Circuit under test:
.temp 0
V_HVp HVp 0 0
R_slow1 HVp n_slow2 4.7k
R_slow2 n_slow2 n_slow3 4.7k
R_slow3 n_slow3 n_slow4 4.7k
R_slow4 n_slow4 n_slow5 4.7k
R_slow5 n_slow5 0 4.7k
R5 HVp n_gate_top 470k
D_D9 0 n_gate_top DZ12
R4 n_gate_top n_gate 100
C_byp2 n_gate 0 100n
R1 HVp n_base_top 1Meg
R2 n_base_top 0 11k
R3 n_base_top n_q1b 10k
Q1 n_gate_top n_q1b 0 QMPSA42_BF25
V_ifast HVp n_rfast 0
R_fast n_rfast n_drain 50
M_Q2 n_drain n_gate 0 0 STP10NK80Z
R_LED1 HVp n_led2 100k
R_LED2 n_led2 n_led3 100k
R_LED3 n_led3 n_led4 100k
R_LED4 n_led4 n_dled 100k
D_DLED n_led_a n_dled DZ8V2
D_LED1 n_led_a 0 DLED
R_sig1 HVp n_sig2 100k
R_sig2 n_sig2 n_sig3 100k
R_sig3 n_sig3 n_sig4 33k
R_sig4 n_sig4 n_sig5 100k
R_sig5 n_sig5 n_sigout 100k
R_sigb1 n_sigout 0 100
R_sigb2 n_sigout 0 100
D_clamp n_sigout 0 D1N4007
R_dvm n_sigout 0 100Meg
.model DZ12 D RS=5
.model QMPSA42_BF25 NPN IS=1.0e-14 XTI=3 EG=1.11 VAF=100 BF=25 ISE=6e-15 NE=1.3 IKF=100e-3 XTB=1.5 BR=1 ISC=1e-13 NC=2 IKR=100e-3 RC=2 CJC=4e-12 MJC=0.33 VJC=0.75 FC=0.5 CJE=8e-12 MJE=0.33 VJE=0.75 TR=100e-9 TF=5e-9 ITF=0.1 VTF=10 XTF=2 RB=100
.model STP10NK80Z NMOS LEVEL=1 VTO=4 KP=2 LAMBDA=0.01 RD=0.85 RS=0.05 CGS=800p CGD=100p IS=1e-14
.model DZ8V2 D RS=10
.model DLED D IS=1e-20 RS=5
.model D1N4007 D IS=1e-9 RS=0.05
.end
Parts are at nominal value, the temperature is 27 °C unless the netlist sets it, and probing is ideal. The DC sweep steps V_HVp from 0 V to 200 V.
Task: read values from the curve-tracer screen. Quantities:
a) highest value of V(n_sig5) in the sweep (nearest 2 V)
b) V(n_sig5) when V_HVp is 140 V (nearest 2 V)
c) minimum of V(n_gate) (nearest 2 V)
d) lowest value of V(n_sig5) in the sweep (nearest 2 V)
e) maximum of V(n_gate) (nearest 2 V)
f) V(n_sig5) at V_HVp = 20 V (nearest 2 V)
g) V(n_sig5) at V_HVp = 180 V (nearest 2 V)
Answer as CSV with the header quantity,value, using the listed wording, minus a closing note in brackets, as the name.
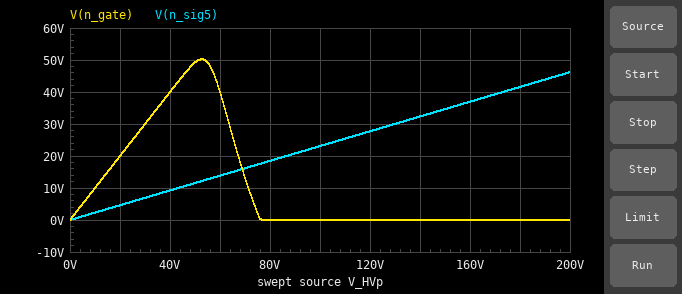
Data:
quantity,value
highest value of V(n_sig5) in the sweep,46 V
V(n_sig5) when V_HVp is 140 V,32 V
minimum of V(n_gate),0 V
lowest value of V(n_sig5) in the sweep,0 V
maximum of V(n_gate),50 V
V(n_sig5) at V_HVp = 20 V,4 V
V(n_sig5) at V_HVp = 180 V,42 V
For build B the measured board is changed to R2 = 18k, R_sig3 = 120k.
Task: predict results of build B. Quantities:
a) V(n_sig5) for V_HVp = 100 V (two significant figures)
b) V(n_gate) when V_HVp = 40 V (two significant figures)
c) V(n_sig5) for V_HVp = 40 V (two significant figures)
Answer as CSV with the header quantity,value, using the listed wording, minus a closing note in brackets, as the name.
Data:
quantity,value
V(n_sig5) for V_HVp = 100 V,19 V
V(n_gate) when V_HVp = 40 V,12 V
V(n_sig5) for V_HVp = 40 V,7.7 V
